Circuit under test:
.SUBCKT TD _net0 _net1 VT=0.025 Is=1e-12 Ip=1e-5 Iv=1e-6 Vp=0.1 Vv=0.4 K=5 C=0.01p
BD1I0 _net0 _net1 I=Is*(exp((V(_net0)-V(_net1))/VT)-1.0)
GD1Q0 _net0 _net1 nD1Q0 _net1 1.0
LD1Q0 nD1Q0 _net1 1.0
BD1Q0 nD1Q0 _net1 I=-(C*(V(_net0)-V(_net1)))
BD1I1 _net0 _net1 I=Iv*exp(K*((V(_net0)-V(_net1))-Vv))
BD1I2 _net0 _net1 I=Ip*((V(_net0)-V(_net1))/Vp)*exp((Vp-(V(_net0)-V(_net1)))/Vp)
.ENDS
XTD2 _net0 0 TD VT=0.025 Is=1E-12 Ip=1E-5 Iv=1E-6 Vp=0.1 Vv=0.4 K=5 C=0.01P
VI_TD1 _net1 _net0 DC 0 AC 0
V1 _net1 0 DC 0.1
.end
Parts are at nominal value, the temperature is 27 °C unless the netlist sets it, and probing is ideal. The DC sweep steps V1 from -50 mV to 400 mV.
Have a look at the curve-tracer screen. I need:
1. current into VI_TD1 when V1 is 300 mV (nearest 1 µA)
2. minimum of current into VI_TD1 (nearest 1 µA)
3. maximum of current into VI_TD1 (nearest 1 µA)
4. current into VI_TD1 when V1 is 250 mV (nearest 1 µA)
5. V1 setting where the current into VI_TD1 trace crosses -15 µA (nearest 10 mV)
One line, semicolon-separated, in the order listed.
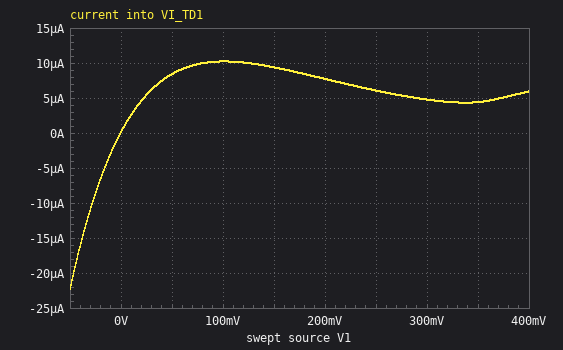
5 µA; -22 µA; 10 µA; 6 µA; -40 mV
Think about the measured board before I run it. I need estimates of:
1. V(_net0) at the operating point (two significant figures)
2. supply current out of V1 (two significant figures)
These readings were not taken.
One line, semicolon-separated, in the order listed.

100 mV; 10 µA
